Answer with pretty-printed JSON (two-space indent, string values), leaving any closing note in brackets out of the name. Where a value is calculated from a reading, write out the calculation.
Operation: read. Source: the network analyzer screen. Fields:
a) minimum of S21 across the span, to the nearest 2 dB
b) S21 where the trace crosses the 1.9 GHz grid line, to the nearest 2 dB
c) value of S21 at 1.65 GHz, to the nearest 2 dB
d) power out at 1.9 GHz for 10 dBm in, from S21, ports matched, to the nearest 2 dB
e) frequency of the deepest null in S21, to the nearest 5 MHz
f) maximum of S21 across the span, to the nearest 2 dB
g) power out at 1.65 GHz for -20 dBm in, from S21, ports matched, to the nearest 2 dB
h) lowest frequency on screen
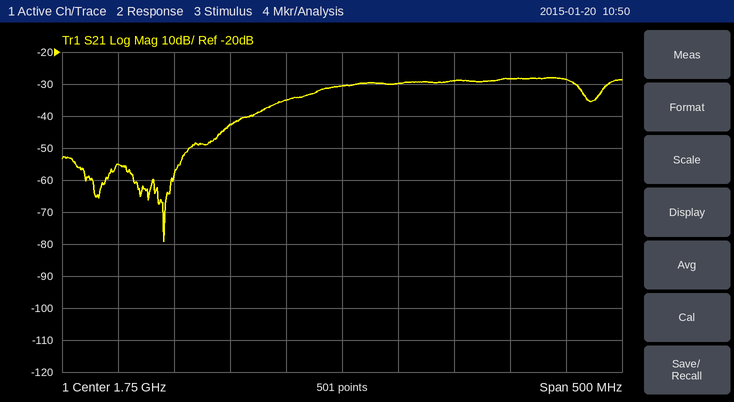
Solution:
{
  "minimum of S21 across the span, to the nearest 2 dB": "-80 dB",
  "S21 where the trace crosses the 1.9 GHz grid line, to the nearest 2 dB": "-28 dB",
  "value of S21 at 1.65 GHz, to the nearest 2 dB": "-42 dB",
  "power out at 1.9 GHz for 10 dBm in, from S21, ports matched, to the nearest 2 dB": "10 dBm + (-28 dB) = -18 dBm",
  "frequency of the deepest null in S21, to the nearest 5 MHz": "1.590 GHz",
  "maximum of S21 across the span, to the nearest 2 dB": "-28 dB",
  "power out at 1.65 GHz for -20 dBm in, from S21, ports matched, to the nearest 2 dB": "-20 dBm + (-42 dB) = -62 dBm",
  "lowest frequency on screen": "1.5 GHz"
}
